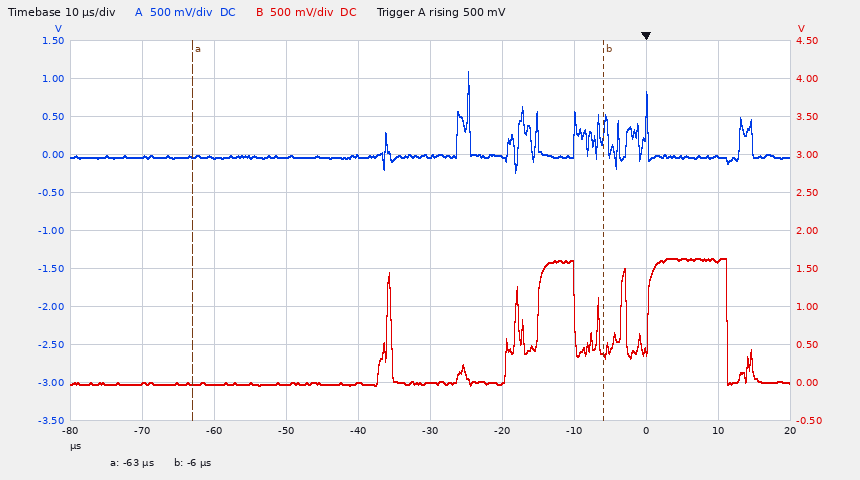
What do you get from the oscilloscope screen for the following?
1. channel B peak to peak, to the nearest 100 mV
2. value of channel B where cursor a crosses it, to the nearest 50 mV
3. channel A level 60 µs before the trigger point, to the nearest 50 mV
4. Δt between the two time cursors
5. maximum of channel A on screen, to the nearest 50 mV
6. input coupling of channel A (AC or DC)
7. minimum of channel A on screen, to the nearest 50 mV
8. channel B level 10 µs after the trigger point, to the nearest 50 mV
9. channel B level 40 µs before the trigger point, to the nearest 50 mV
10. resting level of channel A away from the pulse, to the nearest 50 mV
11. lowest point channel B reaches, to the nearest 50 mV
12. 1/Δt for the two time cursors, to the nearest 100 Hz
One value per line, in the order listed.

1.70 V
0 mV
-50 mV
57 µs
1.10 V
DC
-250 mV
1.60 V
0 mV
-50 mV
-50 mV
17.5 kHz
